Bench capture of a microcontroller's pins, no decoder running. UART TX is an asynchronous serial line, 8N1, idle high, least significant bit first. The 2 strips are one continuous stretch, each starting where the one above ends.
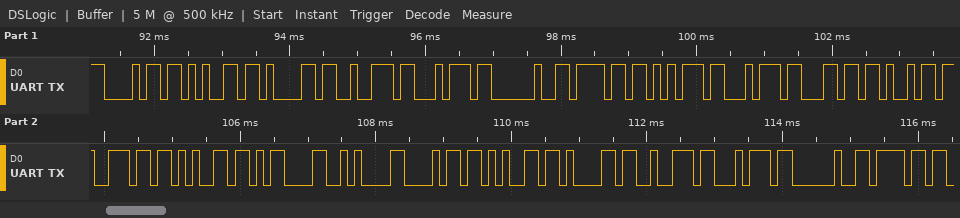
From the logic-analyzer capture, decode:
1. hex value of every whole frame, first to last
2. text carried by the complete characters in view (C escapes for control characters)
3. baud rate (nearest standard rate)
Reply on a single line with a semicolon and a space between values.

68 65 61 72 74 20 6F 75 74 6C 69 6E 65 0D 0A 68 65 61 72 74 20 6F; "heart outline\r\nheart o"; 9600 baud
